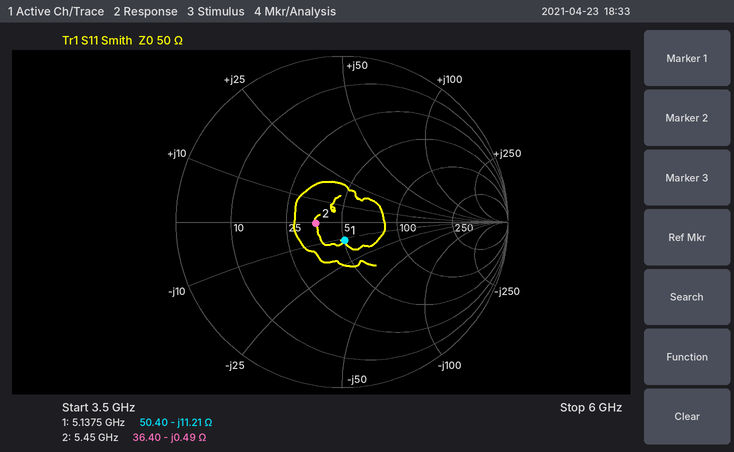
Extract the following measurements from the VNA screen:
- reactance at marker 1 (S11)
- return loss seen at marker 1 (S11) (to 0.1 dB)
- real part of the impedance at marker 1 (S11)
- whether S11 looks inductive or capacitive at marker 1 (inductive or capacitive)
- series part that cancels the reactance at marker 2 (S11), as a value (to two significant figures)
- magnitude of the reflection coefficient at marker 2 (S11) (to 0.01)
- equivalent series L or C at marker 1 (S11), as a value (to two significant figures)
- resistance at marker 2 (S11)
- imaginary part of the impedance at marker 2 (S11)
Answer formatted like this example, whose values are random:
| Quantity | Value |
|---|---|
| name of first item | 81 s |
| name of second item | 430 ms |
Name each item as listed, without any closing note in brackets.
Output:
| Quantity | Value |
|---|---|
| reactance at marker 1 | -11.21 Ω |
| return loss seen at marker 1 (S11) | 19.1 dB |
| real part of the impedance at marker 1 | 50.40 Ω |
| whether S11 looks inductive or capacitive at marker 1 | capacitive |
| series part that cancels the reactance at marker 2 (S11), as a value | 14 pH |
| magnitude of the reflection coefficient at marker 2 (S11) | 0.16 |
| equivalent series L or C at marker 1 (S11), as a value | 2.8 pF |
| resistance at marker 2 | 36.40 Ω |
| imaginary part of the impedance at marker 2 | -0.49 Ω |
